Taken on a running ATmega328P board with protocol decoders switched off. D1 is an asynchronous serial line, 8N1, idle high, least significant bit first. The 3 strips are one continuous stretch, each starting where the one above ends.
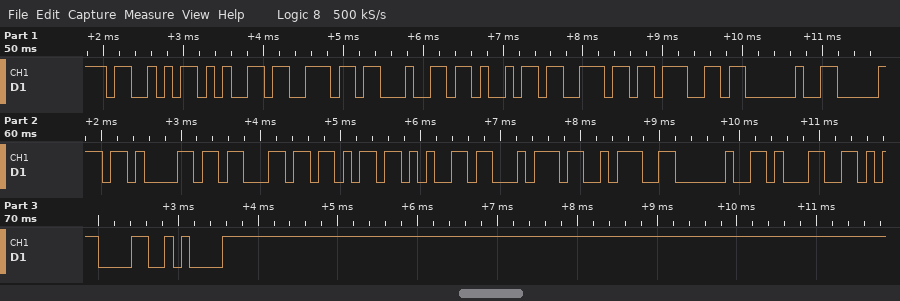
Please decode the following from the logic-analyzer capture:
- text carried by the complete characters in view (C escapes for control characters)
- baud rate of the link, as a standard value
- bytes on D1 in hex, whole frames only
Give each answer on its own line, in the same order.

"Sending packet: 1\r\n"
9600 baud
53 65 6E 64 69 6E 67 20 70 61 63 6B 65 74 3A 20 31 0D 0A
